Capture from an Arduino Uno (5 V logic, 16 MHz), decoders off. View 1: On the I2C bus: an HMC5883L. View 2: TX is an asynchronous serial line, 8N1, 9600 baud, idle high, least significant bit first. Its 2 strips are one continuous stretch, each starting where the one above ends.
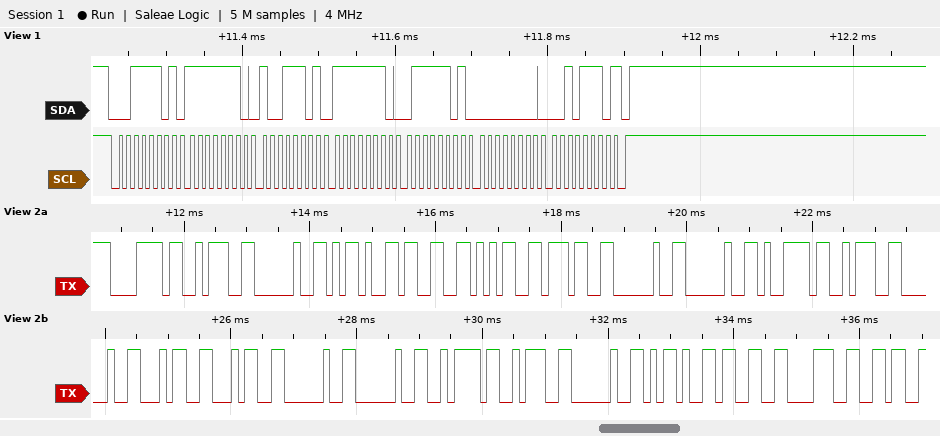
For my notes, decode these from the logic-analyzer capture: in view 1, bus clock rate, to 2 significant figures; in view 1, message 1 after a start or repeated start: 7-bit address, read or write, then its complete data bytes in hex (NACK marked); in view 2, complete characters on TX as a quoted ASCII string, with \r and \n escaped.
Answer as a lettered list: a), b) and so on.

a) 100 kHz
b) 0x1E read: FE 9D FE 7D 00 2E NACK
c) "x: -357  y: 44  z: -386"
